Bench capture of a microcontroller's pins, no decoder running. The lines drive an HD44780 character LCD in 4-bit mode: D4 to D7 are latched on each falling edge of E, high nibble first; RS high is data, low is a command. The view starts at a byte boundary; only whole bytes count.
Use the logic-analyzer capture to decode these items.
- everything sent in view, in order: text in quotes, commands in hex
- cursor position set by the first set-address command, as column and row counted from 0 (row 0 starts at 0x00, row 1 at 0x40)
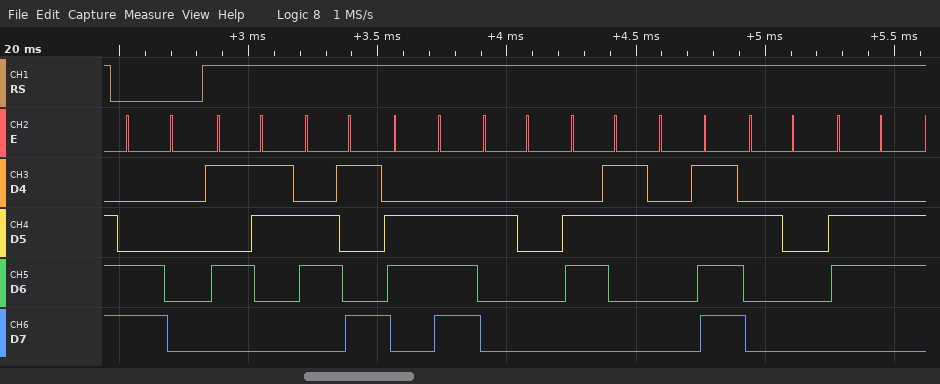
0xC0 "Sin c/ f"
column 0, row 1
